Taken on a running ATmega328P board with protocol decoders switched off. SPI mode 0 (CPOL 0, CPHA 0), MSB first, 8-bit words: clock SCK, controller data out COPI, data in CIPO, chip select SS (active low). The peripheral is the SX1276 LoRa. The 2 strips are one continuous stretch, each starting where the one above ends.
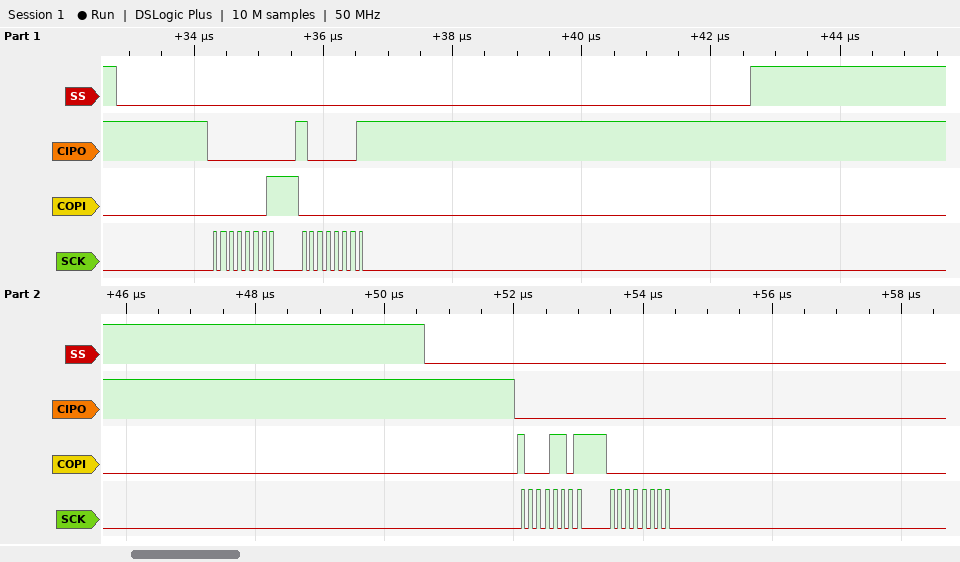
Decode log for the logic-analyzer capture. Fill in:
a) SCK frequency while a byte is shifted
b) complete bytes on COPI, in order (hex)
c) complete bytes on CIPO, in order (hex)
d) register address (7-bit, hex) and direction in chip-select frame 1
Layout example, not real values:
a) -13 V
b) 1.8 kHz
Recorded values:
a) 8 MHz
b) 0x01 0x00 0x8D 0x00
c) 0x00 0x81 0x00 0x00
d) 0x01 read
